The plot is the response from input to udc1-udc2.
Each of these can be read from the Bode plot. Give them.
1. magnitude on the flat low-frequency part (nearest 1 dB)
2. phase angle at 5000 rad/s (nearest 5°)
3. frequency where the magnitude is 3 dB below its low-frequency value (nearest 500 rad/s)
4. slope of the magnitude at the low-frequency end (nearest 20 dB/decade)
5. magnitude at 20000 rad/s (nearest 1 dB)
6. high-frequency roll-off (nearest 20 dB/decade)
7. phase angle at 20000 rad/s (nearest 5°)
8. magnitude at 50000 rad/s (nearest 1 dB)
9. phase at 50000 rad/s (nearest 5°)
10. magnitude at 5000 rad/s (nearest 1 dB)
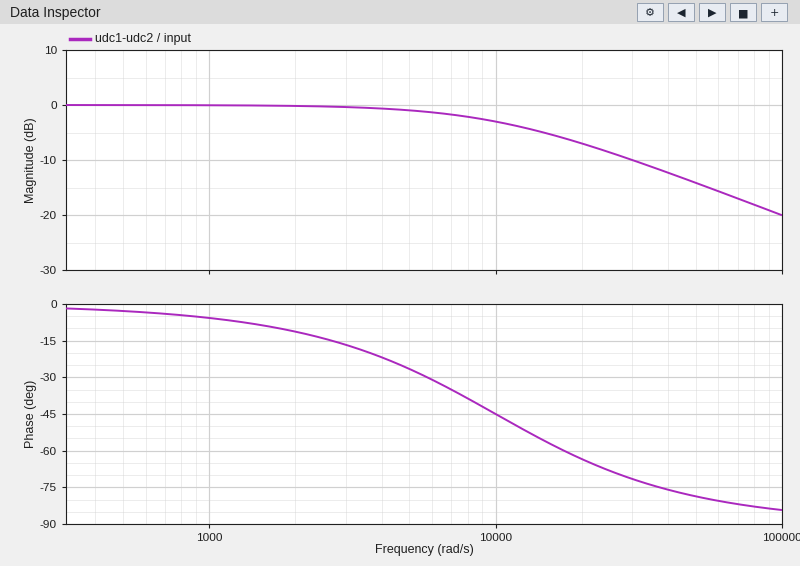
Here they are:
0 dB
-25°
10000 rad/s
0 dB/decade
-7 dB
-20 dB/decade
-65°
-14 dB
-80°
-1 dB
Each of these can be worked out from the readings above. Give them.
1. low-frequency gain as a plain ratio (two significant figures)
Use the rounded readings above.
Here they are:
1.0
